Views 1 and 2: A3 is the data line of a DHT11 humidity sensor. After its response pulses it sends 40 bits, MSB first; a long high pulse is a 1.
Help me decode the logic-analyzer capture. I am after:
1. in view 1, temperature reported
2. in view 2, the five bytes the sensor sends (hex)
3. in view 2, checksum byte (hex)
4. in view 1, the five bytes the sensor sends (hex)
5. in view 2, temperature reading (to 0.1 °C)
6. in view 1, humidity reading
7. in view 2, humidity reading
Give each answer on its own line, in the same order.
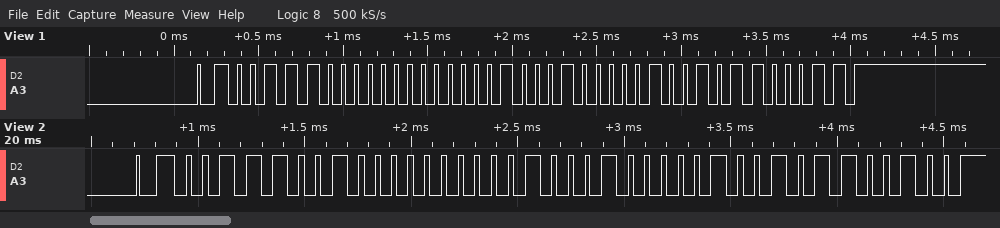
34.9 °C
39 00 22 09 64
0x64
38 00 22 09 63
34.9 °C
56 %
57 %
